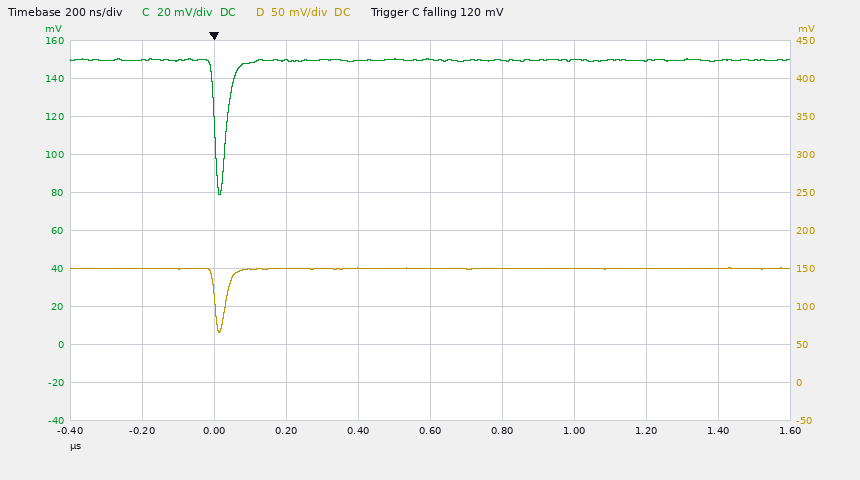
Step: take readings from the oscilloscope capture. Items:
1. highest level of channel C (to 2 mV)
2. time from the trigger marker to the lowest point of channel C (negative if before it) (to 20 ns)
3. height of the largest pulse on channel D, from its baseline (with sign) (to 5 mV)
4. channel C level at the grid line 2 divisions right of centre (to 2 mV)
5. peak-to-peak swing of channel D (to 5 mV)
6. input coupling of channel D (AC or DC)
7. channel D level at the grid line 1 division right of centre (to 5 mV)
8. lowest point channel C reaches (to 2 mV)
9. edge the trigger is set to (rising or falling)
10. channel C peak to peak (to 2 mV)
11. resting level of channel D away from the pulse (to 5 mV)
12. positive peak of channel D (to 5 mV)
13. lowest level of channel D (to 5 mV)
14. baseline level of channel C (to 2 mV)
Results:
150 mV
+20 ns
-85 mV
150 mV
85 mV
DC
150 mV
78 mV
falling
72 mV
150 mV
150 mV
65 mV
150 mV
